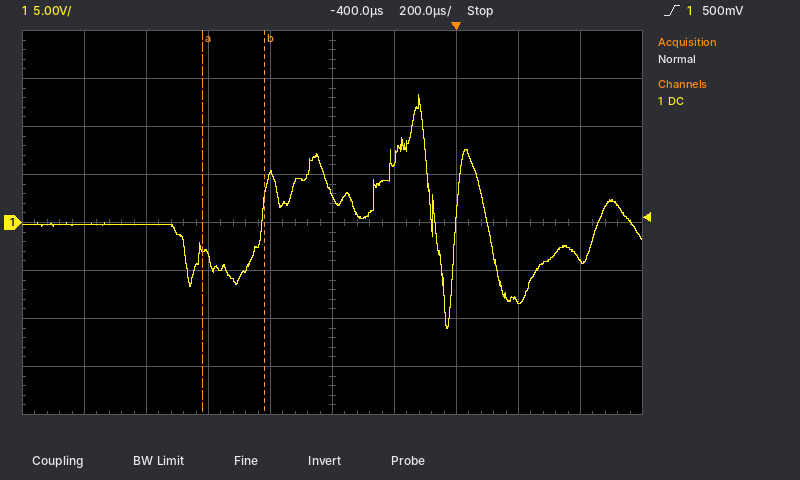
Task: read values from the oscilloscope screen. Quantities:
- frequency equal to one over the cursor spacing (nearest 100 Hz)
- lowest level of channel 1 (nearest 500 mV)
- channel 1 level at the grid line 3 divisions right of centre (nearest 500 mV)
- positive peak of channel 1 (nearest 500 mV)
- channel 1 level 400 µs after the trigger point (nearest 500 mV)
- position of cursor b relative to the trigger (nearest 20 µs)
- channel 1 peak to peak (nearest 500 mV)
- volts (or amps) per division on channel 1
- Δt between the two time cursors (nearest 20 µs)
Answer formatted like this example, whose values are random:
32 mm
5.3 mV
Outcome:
5.0 kHz
-11.0 V
-8.0 V
13.5 V
-4.0 V
-620 µs
24.5 V
5 V
200 µs
